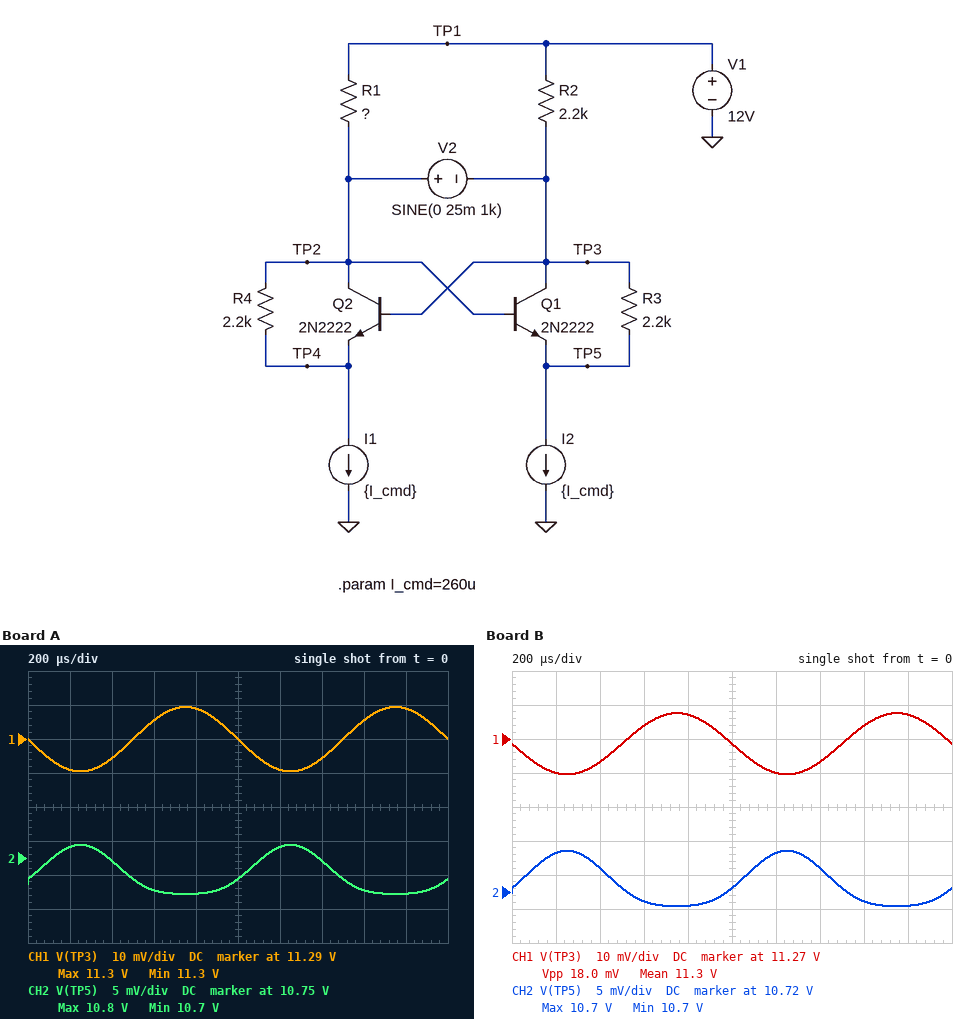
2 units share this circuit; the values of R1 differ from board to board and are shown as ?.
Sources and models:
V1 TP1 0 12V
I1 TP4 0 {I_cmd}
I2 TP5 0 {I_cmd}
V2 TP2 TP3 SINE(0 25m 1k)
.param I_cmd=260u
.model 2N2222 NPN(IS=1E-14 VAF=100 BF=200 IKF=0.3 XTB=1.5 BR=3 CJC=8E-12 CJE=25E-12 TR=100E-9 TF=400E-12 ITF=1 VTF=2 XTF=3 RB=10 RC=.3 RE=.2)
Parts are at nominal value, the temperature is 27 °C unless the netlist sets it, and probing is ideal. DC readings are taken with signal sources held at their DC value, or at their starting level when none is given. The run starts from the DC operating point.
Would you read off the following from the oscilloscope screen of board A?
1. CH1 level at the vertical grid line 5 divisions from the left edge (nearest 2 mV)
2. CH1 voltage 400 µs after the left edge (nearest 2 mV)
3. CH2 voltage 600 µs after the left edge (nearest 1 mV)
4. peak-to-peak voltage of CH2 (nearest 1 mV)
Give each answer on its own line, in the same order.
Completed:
11.290 V
11.284 V
10.745 V
7 mV
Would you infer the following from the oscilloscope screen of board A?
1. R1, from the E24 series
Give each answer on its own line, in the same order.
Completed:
3.6 kΩ
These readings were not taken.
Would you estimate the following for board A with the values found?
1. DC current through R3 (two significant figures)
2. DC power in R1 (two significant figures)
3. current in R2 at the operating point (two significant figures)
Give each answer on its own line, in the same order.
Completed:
250 µA
140 µW
320 µA
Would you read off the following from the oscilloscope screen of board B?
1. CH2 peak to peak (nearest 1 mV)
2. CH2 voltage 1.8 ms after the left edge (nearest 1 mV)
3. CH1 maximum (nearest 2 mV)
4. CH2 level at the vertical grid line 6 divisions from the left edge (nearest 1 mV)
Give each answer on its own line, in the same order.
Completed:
8 mV
10.723 V
11.278 V
10.731 V
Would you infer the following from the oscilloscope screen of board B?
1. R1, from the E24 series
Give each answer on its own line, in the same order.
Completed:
3.9 kΩ
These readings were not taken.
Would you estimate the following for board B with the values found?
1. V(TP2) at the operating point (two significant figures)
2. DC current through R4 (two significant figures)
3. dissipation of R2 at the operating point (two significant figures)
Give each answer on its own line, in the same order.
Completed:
11 V
250 µA
240 µW
